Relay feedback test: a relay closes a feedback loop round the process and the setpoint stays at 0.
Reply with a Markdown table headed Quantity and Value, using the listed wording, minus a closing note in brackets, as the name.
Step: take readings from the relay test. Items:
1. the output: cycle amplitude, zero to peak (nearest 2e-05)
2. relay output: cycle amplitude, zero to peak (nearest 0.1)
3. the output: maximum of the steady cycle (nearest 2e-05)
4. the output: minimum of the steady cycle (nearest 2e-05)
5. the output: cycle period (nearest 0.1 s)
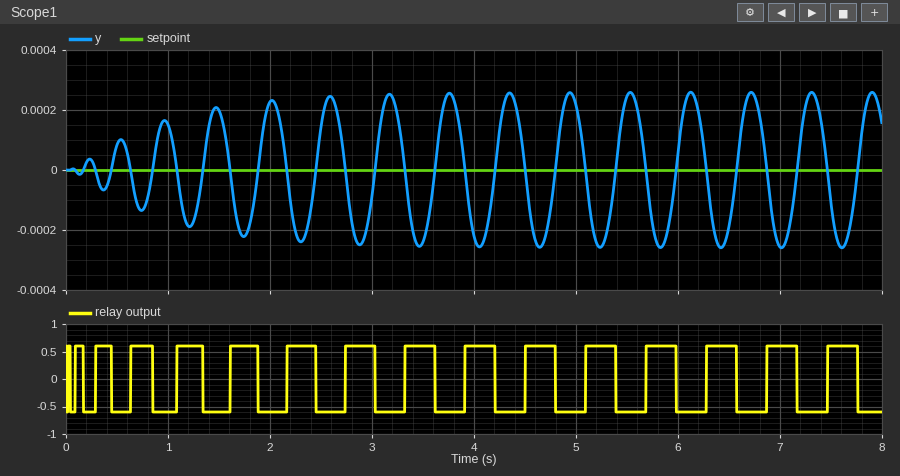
| Quantity | Value |
|---|---|
| the output: cycle amplitude, zero to peak | 0.00026 |
| relay output: cycle amplitude, zero to peak | 0.6 |
| the output: maximum of the steady cycle | 0.00026 |
| the output: minimum of the steady cycle | -0.00026 |
| the output: cycle period | 0.6 s |
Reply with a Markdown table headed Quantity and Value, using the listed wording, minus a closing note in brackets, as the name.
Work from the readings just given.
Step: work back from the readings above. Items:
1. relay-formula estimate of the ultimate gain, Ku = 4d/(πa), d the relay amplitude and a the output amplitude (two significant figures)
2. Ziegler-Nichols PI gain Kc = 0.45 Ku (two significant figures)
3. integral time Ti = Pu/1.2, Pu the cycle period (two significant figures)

| Quantity | Value |
|---|---|
| relay-formula estimate of the ultimate gain, Ku = 4d/(πa), d the relay amplitude and a the output amplitude | 2900 |
| Ziegler-Nichols PI gain Kc = 0.45 Ku | 1300 |
| integral time Ti = Pu/1.2, Pu the cycle period | 0.50 s |
